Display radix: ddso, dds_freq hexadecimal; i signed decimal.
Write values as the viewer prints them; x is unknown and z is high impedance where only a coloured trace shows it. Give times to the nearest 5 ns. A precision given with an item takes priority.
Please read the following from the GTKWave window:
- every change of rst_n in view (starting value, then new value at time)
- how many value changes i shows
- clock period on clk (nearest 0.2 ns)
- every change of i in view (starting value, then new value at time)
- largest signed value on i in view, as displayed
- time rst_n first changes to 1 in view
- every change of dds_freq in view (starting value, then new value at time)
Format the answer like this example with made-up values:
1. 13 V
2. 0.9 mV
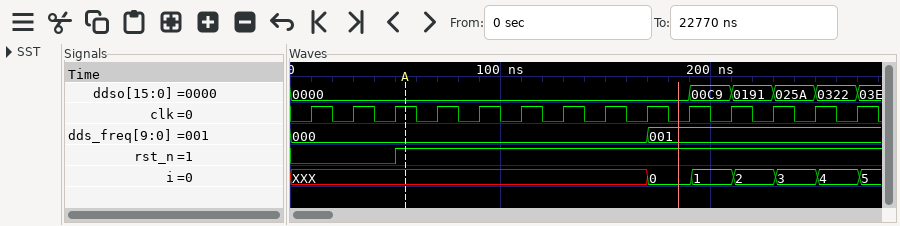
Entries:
1. 0, 1 at 50 ns
2. 6
3. 20 ns
4. XXX, 0 at 170 ns, 1 at 190 ns, 2 at 210 ns, 3 at 230 ns, 4 at 250 ns, 5 at 270 ns
5. 5
6. 50 ns
7. 000, 001 at 170 ns
